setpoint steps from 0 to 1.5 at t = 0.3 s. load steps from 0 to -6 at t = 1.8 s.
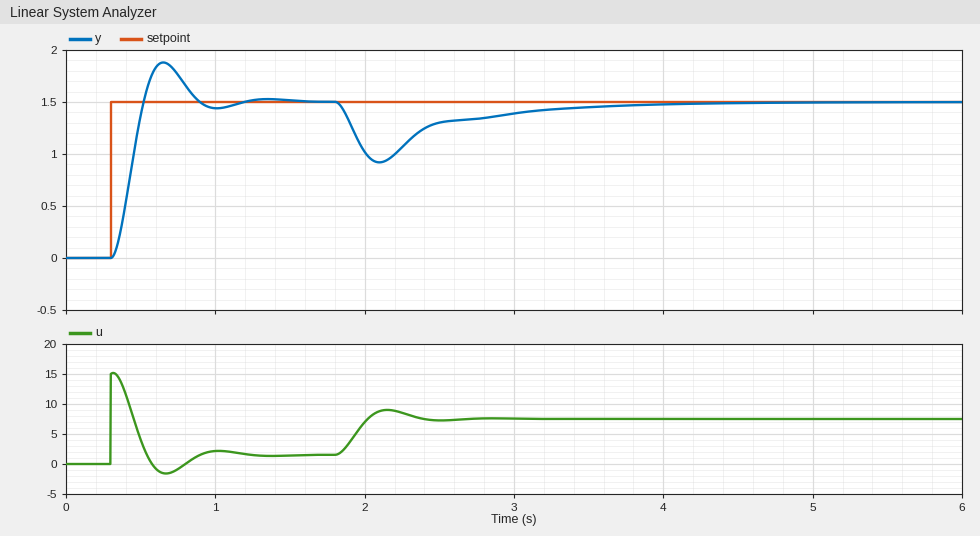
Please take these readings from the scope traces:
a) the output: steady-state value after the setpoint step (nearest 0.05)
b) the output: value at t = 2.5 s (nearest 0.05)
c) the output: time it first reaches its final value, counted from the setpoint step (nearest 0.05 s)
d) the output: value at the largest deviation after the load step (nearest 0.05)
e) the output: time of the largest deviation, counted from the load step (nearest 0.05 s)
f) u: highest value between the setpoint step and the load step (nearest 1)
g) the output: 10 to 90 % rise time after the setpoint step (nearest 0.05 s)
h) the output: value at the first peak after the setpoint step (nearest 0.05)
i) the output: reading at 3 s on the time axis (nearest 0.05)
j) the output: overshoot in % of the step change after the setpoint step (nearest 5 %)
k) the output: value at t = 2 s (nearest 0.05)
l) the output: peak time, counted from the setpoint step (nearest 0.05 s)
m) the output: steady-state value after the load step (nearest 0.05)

1.50
1.30
0.20 s
0.90
0.30 s
15
0.15 s
1.90
1.40
25 %
1.00
0.35 s
1.50
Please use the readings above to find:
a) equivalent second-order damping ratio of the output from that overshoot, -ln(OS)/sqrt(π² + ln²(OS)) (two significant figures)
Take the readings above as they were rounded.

0.40
